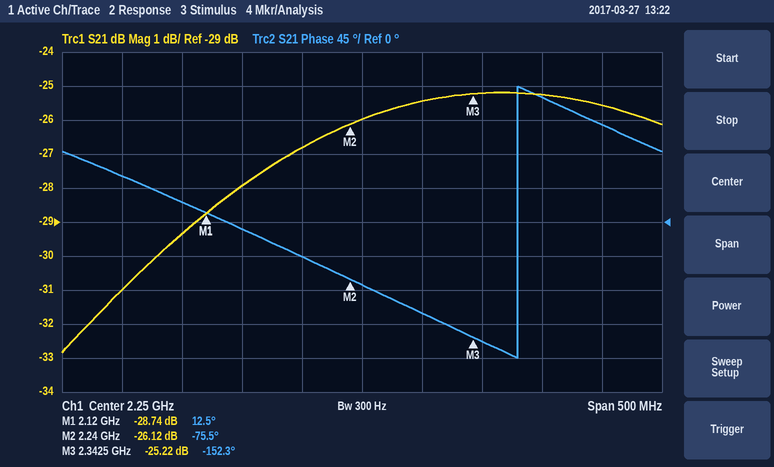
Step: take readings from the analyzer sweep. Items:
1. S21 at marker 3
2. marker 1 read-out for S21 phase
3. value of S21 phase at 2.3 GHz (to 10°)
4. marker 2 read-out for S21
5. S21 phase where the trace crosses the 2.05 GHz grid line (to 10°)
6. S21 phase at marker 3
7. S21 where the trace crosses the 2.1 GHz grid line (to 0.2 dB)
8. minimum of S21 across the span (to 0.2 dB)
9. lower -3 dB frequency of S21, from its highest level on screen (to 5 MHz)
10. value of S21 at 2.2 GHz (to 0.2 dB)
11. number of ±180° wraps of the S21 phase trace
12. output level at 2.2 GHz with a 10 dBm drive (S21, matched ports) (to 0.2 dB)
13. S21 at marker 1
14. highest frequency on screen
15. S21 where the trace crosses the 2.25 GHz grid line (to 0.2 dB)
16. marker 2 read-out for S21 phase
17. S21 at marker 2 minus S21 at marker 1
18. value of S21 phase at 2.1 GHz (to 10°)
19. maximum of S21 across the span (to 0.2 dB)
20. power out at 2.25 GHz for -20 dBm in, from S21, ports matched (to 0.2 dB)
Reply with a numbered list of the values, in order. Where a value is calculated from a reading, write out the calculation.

1. -25.22 dB
2. 12.5°
3. -120°
4. -26.12 dB
5. 60°
6. -152.3°
7. -29.4 dB
8. -32.8 dB
9. 2.140 GHz
10. -26.8 dB
11. 1
12. 10 dBm + (-26.8 dB) = -16.8 dBm
13. -28.74 dB
14. 2.5 GHz
15. -26.0 dB
16. -75.5°
17. -26.12 − (-28.74) = 2.62 dB
18. 30°
19. -25.2 dB
20. -20 dBm + (-26.0 dB) = -46.0 dBm
